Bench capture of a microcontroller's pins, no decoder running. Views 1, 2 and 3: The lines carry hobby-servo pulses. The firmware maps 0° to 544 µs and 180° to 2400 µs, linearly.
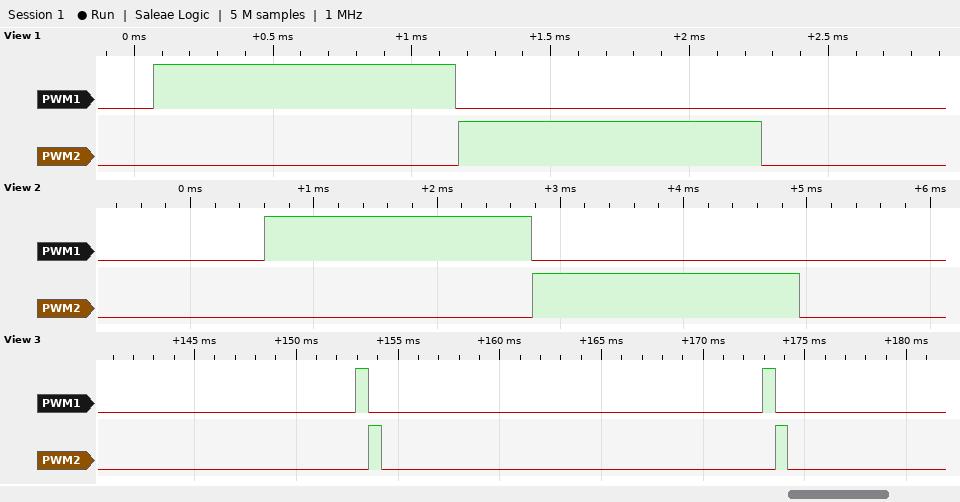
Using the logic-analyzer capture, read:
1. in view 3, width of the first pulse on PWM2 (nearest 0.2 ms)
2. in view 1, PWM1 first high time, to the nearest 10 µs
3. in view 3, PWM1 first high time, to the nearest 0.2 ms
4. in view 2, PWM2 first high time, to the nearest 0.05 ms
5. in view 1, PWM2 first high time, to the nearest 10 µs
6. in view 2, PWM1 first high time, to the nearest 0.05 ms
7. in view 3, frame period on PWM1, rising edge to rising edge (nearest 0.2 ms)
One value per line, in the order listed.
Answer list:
0.6 ms
1090 µs
0.6 ms
2.15 ms
1090 µs
2.15 ms
20.0 ms
